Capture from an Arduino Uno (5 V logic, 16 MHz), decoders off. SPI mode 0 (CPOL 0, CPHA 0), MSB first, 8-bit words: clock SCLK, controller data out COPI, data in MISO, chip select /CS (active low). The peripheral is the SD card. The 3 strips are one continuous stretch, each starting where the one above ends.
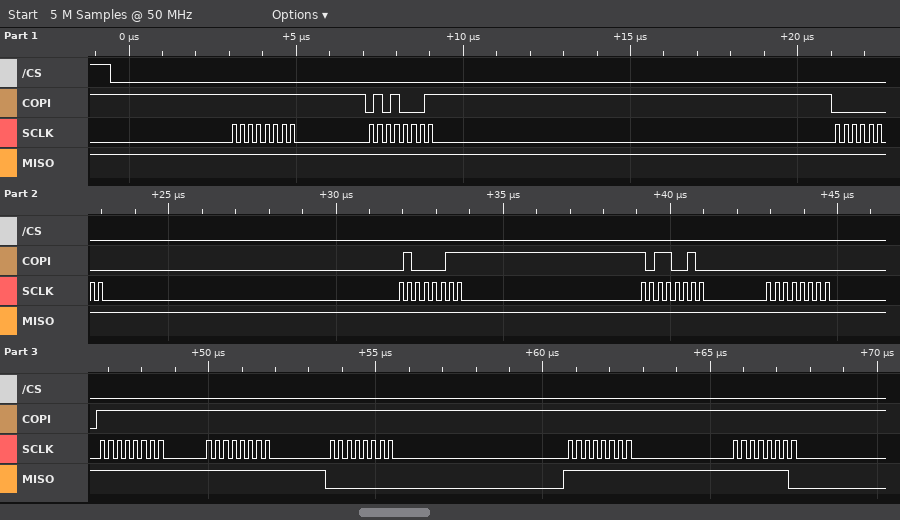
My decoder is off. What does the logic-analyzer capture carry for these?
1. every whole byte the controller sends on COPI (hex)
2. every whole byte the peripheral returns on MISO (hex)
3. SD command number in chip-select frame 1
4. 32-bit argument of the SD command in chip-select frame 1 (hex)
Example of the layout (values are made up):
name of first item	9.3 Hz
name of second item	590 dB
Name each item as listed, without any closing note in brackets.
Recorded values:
every whole byte the controller sends on COPI	0xFF 0x51 0x00 0x43 0xB2 0x00 0xFF 0xFF 0xFF 0xFF 0xFF
every whole byte the peripheral returns on MISO	0xFF 0xFF 0xFF 0xFF 0xFF 0xFF 0xFF 0xFF 0x00 0xFF 0xFE
SD command number in chip-select frame 1	CMD17
32-bit argument of the SD command in chip-select frame 1	0x0043B200
